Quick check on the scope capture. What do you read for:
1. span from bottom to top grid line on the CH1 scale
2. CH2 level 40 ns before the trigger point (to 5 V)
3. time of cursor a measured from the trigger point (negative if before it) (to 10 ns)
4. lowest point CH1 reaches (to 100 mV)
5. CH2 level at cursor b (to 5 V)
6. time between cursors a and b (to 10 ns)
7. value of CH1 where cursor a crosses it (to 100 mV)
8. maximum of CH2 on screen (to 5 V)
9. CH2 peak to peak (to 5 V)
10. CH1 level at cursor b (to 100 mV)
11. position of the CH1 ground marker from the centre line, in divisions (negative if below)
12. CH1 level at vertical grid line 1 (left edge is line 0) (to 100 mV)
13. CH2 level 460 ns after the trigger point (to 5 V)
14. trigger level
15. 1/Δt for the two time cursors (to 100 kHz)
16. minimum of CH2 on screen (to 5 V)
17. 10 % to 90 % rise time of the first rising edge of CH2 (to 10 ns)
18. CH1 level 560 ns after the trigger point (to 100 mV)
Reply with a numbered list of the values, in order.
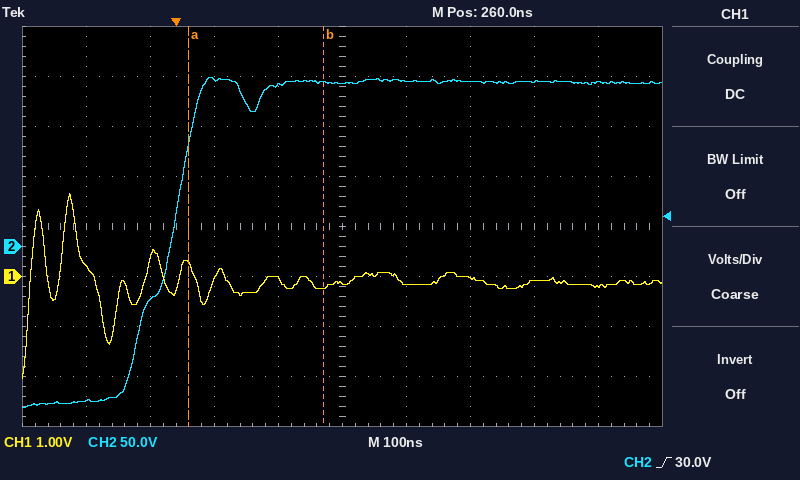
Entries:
1. 8 V
2. -55 V
3. +20 ns
4. -2.0 V
5. 165 V
6. 210 ns
7. 200 mV
8. 170 V
9. 330 V
10. -200 mV
11. -1.0 div
12. 200 mV
13. 165 V
14. 30.0 V
15. 4.8 MHz
16. -160 V
17. 100 ns
18. -100 mV
